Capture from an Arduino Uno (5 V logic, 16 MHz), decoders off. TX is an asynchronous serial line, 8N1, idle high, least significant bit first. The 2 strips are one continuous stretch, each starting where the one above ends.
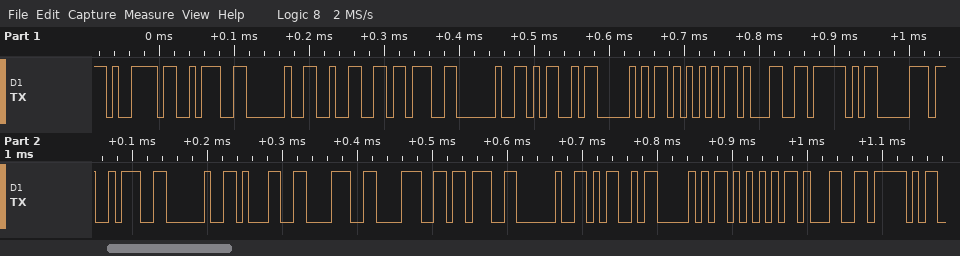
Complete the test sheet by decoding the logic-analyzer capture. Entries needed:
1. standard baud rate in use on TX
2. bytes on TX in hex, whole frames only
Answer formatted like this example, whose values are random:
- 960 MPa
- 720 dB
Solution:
- 115200 baud
- 0x79 0x3A 0x20 0x32 0x3B 0x20 0x4D 0x50 0x55 0x31 0x5F 0x70 0x3A 0x20 0x31 0x38 0x38 0x3B 0x20 0x4D 0x50 0x55 0x31 0x5F
